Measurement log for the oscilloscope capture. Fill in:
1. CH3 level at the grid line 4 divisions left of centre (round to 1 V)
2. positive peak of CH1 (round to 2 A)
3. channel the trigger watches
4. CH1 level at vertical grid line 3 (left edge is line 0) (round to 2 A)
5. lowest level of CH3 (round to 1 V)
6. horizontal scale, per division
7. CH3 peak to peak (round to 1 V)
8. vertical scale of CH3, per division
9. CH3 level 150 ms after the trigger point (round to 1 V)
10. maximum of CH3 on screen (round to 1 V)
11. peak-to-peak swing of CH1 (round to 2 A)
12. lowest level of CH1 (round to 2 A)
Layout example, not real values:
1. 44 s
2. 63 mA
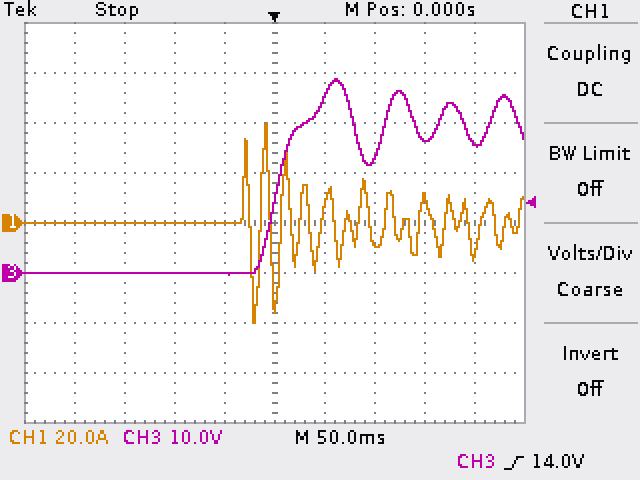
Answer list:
1. 0 V
2. 40 A
3. CH3
4. 0 A
5. 0 V
6. 50 ms
7. 39 V
8. 10 V
9. 27 V
10. 39 V
11. 80 A
12. -40 A
